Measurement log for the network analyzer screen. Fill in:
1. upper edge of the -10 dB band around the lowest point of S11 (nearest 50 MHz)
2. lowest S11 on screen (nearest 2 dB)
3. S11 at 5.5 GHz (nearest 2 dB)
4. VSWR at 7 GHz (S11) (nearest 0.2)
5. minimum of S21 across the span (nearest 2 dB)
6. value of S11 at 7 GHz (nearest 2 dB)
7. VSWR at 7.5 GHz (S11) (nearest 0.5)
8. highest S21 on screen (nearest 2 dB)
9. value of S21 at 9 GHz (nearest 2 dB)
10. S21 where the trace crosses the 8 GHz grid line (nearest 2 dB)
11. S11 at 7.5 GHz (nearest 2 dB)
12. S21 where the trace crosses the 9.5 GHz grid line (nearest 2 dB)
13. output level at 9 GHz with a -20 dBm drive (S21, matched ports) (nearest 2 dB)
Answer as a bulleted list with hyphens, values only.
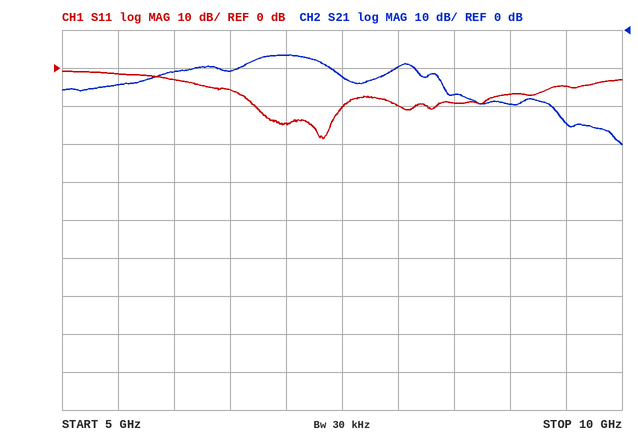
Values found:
- 7.50 GHz
- -18 dB
- -2 dB
- 1.4
- -30 dB
- -14 dB
- 2.0
- -6 dB
- -20 dB
- -10 dB
- -10 dB
- -24 dB
- -40 dBm
